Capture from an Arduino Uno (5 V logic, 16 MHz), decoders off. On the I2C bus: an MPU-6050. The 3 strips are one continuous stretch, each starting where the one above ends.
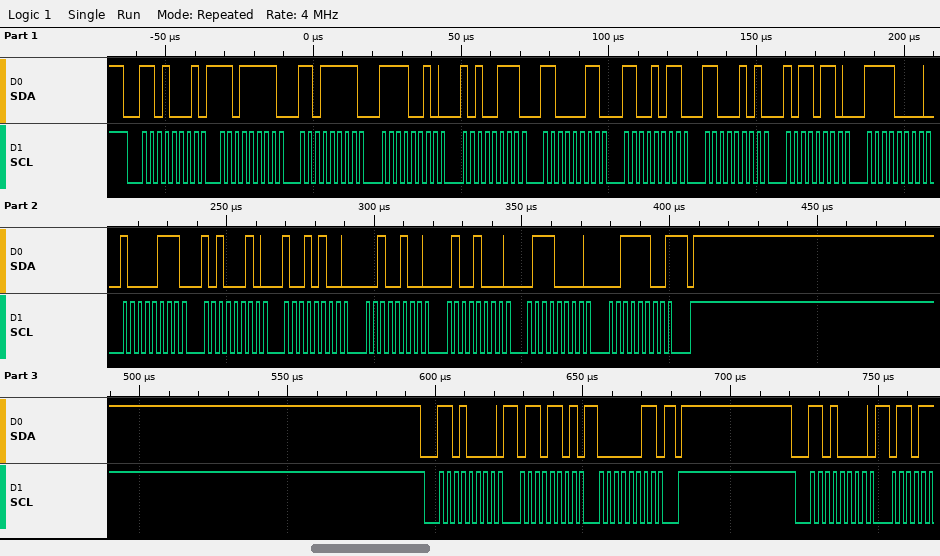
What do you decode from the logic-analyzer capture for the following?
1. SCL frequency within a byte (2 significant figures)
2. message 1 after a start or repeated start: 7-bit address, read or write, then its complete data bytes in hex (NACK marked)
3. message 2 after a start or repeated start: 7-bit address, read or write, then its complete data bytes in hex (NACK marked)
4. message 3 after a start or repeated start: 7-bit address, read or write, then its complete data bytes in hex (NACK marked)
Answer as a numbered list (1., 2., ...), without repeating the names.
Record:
1. 400 kHz
2. 0x68 read: DF DF F2 A7 C3 CB C5 B6 F0 87 A2 94 24 48 70 3C NACK
3. 0x68 write: 6D 03
4. 0x68 write
